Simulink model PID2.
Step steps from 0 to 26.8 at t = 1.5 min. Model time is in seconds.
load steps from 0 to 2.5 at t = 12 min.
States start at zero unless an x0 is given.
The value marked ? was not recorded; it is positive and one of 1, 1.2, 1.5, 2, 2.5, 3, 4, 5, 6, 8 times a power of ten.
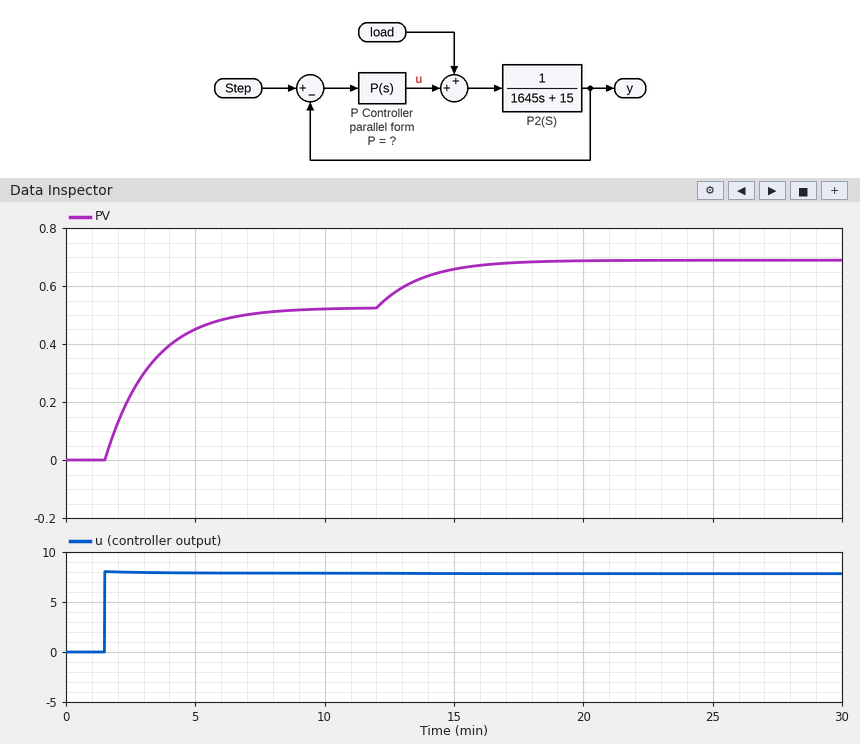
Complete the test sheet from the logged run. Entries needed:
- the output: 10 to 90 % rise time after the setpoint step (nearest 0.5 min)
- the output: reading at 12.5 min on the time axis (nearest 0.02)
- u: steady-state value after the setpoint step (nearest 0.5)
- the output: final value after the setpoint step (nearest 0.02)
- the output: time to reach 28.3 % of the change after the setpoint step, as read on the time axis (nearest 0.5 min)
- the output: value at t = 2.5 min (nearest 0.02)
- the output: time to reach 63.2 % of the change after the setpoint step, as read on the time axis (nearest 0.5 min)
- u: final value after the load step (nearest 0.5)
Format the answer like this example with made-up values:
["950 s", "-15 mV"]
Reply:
["4.0 min", "0.56", "8.0", "0.52", "2.0 min", "0.22", "3.5 min", "8.0"]
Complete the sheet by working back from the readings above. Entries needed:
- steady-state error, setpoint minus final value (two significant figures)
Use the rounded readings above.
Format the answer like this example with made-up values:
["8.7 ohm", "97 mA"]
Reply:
["26"]
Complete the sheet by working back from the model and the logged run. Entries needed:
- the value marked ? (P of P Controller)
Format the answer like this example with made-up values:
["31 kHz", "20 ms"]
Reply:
["0.3"]
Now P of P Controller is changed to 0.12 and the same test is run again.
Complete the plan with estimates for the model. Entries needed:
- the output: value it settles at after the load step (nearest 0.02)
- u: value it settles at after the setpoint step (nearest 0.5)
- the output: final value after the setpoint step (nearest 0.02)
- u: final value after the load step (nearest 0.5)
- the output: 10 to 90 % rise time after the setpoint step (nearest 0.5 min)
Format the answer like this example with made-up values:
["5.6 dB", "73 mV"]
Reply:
["0.38", "3.0", "0.22", "3.0", "4.0 min"]
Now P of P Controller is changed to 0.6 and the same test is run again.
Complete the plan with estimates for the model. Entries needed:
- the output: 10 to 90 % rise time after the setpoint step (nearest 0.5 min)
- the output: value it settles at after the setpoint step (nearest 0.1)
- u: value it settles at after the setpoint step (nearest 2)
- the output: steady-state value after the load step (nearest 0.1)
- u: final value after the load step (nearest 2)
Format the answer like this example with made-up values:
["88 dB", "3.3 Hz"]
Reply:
["4.0 min", "1.0", "16", "1.2", "16"]
